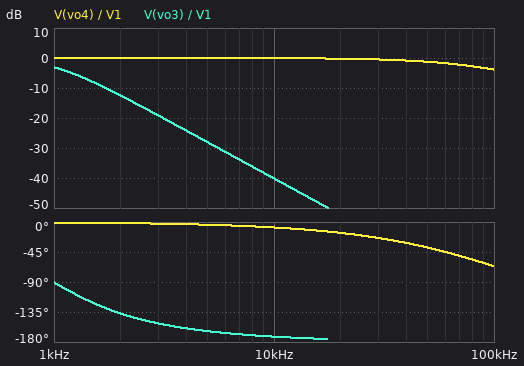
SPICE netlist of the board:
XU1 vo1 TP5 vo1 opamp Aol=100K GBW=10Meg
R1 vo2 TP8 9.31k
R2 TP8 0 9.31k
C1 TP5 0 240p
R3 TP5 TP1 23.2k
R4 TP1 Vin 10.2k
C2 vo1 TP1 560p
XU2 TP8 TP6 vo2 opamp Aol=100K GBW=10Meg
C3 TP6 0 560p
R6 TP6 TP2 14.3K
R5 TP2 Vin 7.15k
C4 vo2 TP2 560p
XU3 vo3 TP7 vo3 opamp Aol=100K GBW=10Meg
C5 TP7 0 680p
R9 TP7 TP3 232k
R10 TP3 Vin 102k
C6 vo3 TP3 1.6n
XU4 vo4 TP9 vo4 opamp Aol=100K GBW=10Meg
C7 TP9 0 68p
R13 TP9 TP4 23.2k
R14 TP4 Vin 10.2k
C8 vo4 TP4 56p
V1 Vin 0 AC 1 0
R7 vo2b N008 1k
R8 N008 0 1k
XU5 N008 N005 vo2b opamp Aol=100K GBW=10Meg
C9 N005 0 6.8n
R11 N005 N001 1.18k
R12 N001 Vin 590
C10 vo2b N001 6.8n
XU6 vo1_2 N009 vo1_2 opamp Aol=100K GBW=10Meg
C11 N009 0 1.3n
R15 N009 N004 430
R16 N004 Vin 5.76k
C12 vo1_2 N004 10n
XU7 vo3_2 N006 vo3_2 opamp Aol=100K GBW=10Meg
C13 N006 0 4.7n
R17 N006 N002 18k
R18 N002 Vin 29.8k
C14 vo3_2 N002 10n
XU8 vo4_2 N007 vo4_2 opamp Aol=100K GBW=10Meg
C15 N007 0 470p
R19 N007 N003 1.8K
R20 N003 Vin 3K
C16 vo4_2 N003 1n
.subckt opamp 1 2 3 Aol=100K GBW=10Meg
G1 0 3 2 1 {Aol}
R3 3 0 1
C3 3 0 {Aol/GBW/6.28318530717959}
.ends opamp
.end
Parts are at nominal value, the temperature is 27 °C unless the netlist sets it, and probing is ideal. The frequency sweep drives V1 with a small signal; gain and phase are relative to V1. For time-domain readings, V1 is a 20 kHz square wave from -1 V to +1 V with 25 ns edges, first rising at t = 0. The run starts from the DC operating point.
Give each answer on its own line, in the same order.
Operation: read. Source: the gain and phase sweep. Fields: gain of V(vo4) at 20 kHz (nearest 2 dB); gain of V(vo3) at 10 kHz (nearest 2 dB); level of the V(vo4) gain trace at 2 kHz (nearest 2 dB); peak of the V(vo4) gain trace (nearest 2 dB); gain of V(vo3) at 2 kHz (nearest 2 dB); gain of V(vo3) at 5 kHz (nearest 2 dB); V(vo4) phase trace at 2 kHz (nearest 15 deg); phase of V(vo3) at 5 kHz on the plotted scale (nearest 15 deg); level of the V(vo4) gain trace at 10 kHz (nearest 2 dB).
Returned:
0 dB
-40 dB
0 dB
0 dB
-12 dB
-28 dB
0 deg
-165 deg
0 dB
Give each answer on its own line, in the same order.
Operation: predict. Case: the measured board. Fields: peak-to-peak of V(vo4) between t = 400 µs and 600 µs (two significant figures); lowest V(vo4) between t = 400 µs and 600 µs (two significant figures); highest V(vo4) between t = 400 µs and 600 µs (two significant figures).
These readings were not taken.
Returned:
2.0 V
-1.0 V
1.0 V
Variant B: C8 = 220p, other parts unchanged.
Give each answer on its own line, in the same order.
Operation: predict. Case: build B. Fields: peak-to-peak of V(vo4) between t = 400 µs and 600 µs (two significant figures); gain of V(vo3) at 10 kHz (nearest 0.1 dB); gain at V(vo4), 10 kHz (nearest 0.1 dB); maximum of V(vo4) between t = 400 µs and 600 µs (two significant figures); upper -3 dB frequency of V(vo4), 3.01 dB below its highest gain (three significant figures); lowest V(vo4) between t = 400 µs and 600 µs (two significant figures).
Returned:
2.4 V
-40.1 dB
0 dB
1.2 V
93.7 kHz
-1.2 V
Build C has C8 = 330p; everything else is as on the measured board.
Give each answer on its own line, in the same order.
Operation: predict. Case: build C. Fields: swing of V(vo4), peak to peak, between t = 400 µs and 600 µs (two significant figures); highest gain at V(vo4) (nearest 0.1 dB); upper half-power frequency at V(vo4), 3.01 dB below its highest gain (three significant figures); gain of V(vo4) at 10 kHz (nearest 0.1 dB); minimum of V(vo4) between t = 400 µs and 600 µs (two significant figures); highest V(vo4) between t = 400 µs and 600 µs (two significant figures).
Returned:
2.7 V
1.4 dB
80.5 kHz
0.1 dB
-1.3 V
1.3 V
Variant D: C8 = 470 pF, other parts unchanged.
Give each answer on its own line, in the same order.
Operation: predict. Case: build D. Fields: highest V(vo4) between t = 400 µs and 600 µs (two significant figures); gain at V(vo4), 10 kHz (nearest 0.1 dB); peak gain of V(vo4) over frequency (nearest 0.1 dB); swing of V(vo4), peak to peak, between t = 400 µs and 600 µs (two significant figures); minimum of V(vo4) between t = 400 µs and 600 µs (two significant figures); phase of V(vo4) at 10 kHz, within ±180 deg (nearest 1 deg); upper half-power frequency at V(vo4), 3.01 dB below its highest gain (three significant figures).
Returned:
1.5 V
0.2 dB
2.5 dB
3.0 V
-1.5 V
-8 deg
68.4 kHz
